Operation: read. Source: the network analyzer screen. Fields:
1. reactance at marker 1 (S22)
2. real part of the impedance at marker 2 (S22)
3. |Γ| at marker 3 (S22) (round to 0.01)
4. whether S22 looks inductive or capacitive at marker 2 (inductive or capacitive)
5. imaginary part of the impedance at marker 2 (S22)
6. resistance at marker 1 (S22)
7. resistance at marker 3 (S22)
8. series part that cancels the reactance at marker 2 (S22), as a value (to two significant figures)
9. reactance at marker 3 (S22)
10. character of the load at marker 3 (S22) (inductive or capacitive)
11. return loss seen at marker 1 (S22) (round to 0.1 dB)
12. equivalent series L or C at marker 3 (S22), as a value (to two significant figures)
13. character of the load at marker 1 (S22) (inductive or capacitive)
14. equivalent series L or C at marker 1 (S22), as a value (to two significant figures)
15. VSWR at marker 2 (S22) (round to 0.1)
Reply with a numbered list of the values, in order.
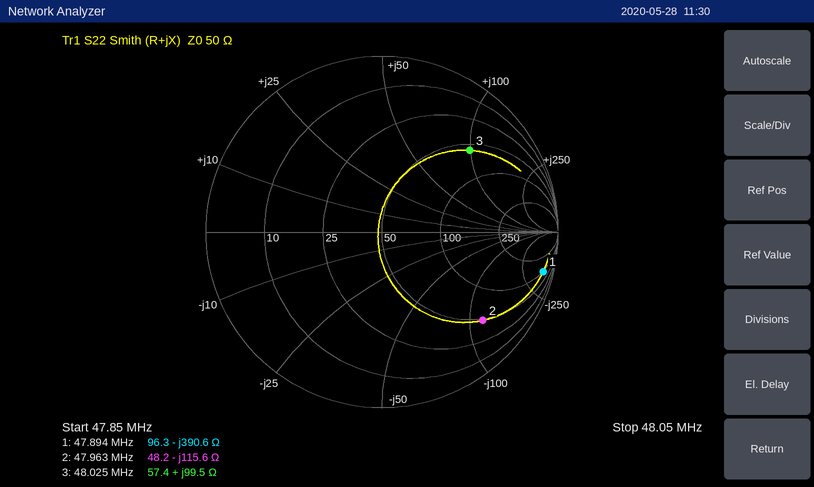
1. -390.6 Ω
2. 48.2 Ω
3. 0.68
4. capacitive
5. -115.6 Ω
6. 96.3 Ω
7. 57.4 Ω
8. 380 nH
9. +99.5 Ω
10. inductive
11. 0.5 dB
12. 330 nH
13. capacitive
14. 8.5 pF
15. 7.4
